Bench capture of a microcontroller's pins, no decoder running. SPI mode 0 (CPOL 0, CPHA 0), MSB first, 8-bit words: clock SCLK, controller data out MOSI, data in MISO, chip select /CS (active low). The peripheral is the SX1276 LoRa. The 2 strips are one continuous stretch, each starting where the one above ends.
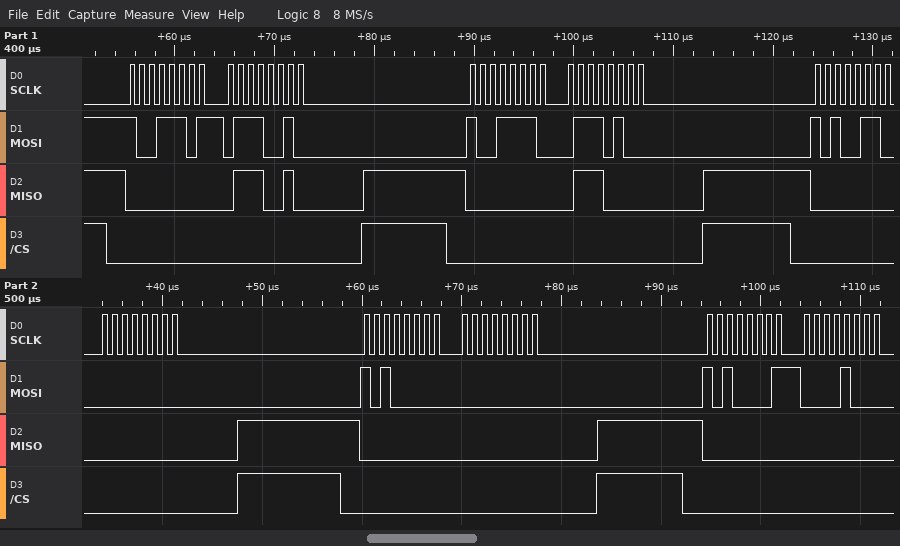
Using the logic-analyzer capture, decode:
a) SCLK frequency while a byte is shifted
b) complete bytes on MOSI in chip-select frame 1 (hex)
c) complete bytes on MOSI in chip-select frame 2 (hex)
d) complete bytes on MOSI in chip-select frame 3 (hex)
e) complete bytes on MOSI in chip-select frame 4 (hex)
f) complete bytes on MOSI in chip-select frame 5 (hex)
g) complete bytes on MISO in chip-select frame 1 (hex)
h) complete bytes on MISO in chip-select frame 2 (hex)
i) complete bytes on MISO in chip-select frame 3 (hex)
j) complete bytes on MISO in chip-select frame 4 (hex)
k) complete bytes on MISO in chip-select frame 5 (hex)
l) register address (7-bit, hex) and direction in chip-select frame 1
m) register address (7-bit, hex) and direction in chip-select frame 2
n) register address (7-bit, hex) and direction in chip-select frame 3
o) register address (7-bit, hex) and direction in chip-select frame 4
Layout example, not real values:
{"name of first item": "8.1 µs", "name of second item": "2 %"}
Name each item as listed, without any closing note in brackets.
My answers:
{"SCLK frequency while a byte is shifted": "1 MHz", "complete bytes on MOSI in chip-select frame 1": "9D 72", "complete bytes on MOSI in chip-select frame 2": "9E 74", "complete bytes on MOSI in chip-select frame 3": "A6 00", "complete bytes on MOSI in chip-select frame 4": "A0 00", "complete bytes on MOSI in chip-select frame 5": "A1 08", "complete bytes on MISO in chip-select frame 1": "00 72", "complete bytes on MISO in chip-select frame 2": "00 70", "complete bytes on MISO in chip-select frame 3": "00 00", "complete bytes on MISO in chip-select frame 4": "00 00", "complete bytes on MISO in chip-select frame 5": "00 00", "register address (7-bit, hex) and direction in chip-select frame 1": "0x1D write", "register address (7-bit, hex) and direction in chip-select frame 2": "0x1E write", "register address (7-bit, hex) and direction in chip-select frame 3": "0x26 write", "register address (7-bit, hex) and direction in chip-select frame 4": "0x20 write"}
